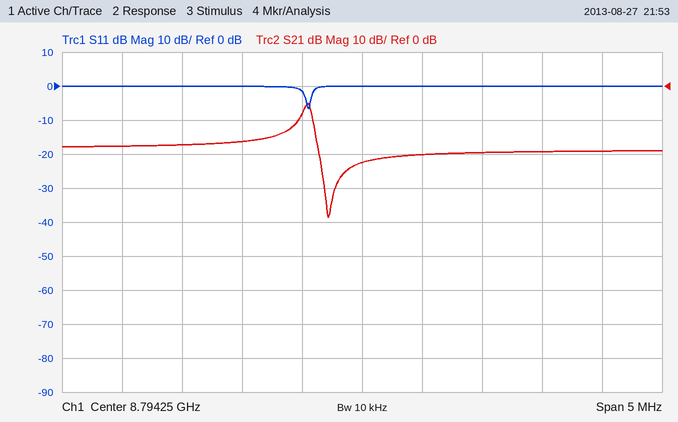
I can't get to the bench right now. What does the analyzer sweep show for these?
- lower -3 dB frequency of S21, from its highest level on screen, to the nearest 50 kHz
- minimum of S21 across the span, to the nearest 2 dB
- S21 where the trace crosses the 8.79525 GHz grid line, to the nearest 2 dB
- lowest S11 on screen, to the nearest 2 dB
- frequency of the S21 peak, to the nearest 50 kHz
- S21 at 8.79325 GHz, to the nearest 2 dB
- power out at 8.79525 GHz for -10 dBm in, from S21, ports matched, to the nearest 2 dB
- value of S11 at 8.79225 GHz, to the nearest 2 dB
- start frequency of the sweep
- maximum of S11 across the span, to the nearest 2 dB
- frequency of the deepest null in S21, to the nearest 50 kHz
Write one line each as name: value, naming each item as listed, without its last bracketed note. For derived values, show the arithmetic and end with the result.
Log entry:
lower -3 dB frequency of S21, from its highest level on screen, to the nearest 50 kHz: 8.79375 GHz
minimum of S21 across the span, to the nearest 2 dB: -38 dB
S21 where the trace crosses the 8.79525 GHz grid line, to the nearest 2 dB: -20 dB
lowest S11 on screen, to the nearest 2 dB: -6 dB
frequency of the S21 peak, to the nearest 50 kHz: 8.79380 GHz
S21 at 8.79325 GHz, to the nearest 2 dB: -16 dB
power out at 8.79525 GHz for -10 dBm in, from S21, ports matched, to the nearest 2 dB: -10 dBm + (-20 dB) = -30 dBm
value of S11 at 8.79225 GHz, to the nearest 2 dB: 0 dB
start frequency of the sweep: 8.79175 GHz
maximum of S11 across the span, to the nearest 2 dB: 0 dB
frequency of the deepest null in S21, to the nearest 50 kHz: 8.79395 GHz
